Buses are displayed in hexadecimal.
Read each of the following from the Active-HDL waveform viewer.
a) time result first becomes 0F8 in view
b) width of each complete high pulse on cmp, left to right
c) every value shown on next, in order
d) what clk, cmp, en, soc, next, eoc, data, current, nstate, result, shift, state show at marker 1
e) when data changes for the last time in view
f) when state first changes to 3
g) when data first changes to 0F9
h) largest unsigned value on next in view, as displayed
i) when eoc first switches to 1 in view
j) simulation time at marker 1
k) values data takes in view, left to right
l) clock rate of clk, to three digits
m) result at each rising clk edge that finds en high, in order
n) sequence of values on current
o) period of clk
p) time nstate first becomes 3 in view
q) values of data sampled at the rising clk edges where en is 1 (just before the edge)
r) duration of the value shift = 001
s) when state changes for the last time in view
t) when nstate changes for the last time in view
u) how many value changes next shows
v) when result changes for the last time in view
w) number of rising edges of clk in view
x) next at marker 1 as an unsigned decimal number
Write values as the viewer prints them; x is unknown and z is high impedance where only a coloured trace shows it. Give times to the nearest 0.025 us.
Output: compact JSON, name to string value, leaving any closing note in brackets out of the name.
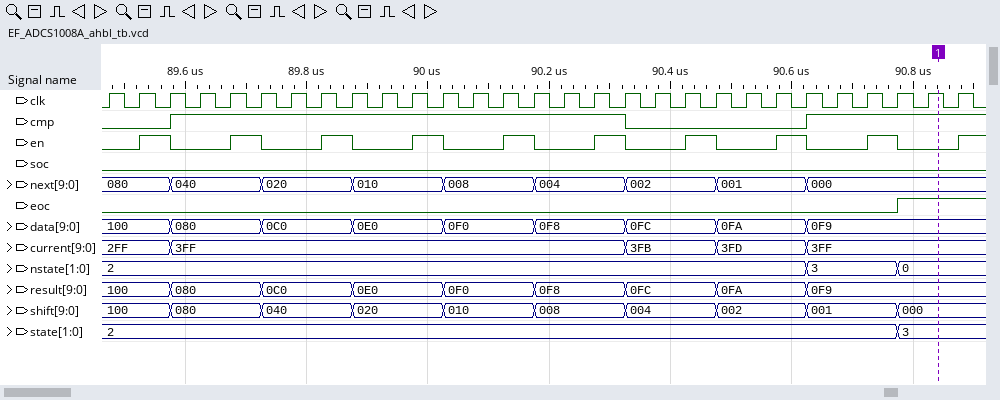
{"time result first becomes 0F8 in view": "90.175 us", "width of each complete high pulse on cmp, left to right": "0.75 us", "every value shown on next, in order": "080, 040, 020, 010, 008, 004, 002, 001, 000", "what clk, cmp, en, soc, next, eoc, data, current, nstate, result, shift, state show at marker 1": "clk=1, cmp=1, en=0, soc=0, next=000, eoc=1, data=0F9, current=3FF, nstate=0, result=0F9, shift=000, state=3", "when data changes for the last time in view": "90.625 us", "when state first changes to 3": "90.775 us", "when data first changes to 0F9": "90.625 us", "largest unsigned value on next in view, as displayed": "080", "when eoc first switches to 1 in view": "90.775 us", "simulation time at marker 1": "90.85 us", "values data takes in view, left to right": "100, 080, 0C0, 0E0, 0F0, 0F8, 0FC, 0FA, 0F9", "clock rate of clk, to three digits": "20.0 MHz", "result at each rising clk edge that finds en high, in order": "100, 080, 0C0, 0E0, 0F0, 0F8, 0FC, 0FA, 0F9", "sequence of values on current": "2FF, 3FF, 3FB, 3FD, 3FF", "period of clk": "0.05 us", "time nstate first becomes 3 in view": "90.625 us", "values of data sampled at the rising clk edges where en is 1": "100, 080, 0C0, 0E0, 0F0, 0F8, 0FC, 0FA, 0F9", "duration of the value shift = 001": "0.15 us", "when state changes for the last time in view": "90.775 us", "when nstate changes for the last time in view": "90.775 us", "how many value changes next shows": "8", "when result changes for the last time in view": "90.625 us", "number of rising edges of clk in view": "29", "next at marker 1 as an unsigned decimal number": "0"}
